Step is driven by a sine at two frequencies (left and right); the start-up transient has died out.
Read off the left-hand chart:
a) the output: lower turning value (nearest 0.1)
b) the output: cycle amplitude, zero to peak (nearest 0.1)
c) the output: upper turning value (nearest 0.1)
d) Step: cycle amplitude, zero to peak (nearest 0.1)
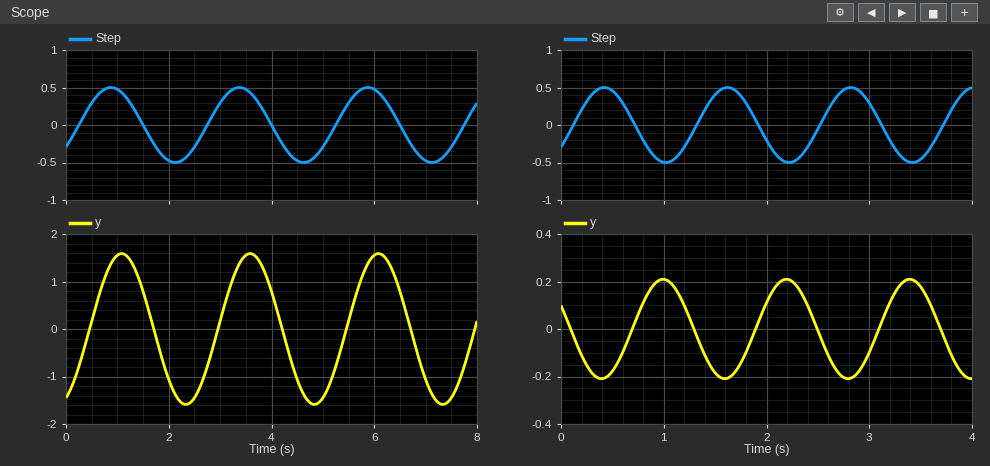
-1.6
1.6
1.6
0.5
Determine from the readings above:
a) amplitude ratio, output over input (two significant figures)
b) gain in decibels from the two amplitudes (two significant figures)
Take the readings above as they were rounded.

3.2
10 dB
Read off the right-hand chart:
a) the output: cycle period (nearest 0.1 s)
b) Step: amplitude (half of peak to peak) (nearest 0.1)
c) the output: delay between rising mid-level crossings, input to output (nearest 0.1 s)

1.2 s
0.5
0.6 s
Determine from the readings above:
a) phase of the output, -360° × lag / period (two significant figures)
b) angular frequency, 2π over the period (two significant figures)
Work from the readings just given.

-180°
5.2 rad/s
